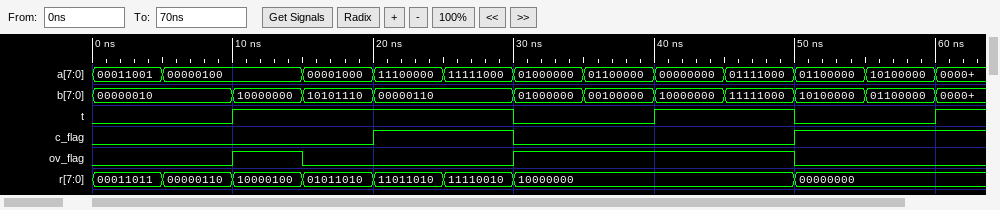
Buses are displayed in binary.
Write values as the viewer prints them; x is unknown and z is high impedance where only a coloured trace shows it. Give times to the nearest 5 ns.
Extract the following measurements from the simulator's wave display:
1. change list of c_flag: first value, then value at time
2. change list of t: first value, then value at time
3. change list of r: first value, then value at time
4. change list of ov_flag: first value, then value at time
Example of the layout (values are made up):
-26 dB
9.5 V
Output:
0, 1 at 20 ns, 0 at 30 ns, 1 at 50 ns
0, 1 at 10 ns, 0 at 30 ns, 1 at 40 ns, 0 at 50 ns, 1 at 60 ns
00011011, 00000110 at 5 ns, 10000100 at 10 ns, 01011010 at 15 ns, 11011010 at 20 ns, 11110010 at 25 ns, 10000000 at 30 ns, 00000000 at 50 ns
0, 1 at 10 ns, 0 at 15 ns, 1 at 30 ns, 0 at 50 ns
